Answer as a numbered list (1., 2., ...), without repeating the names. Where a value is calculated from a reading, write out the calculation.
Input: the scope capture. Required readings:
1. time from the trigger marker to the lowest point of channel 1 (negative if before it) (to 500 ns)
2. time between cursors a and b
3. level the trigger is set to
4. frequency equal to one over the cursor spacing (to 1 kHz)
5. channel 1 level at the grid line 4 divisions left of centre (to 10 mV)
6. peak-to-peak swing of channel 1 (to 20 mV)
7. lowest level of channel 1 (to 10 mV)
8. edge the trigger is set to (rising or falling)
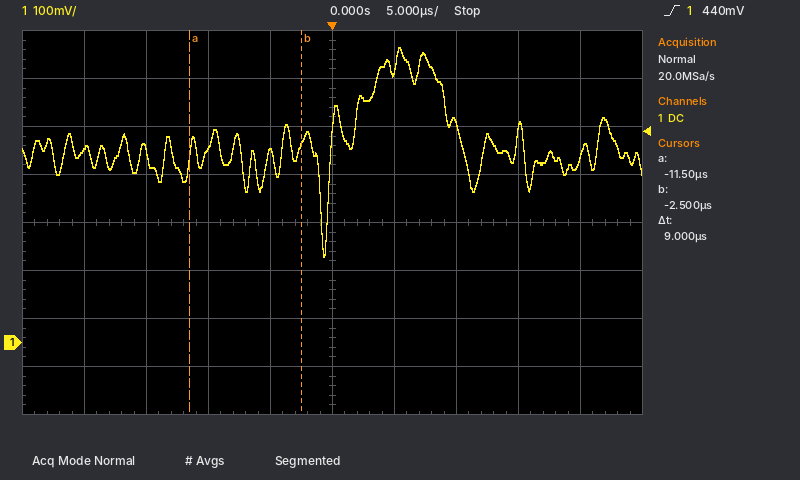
1. -500 ns
2. 9 µs
3. 440 mV
4. 1 / 9 µs ≈ 111 kHz
5. 400 mV
6. 440 mV
7. 180 mV
8. rising
